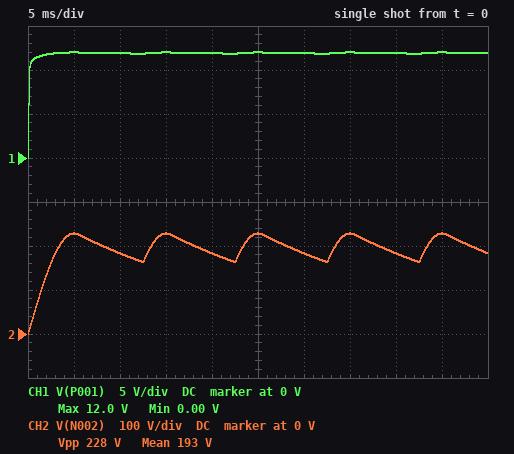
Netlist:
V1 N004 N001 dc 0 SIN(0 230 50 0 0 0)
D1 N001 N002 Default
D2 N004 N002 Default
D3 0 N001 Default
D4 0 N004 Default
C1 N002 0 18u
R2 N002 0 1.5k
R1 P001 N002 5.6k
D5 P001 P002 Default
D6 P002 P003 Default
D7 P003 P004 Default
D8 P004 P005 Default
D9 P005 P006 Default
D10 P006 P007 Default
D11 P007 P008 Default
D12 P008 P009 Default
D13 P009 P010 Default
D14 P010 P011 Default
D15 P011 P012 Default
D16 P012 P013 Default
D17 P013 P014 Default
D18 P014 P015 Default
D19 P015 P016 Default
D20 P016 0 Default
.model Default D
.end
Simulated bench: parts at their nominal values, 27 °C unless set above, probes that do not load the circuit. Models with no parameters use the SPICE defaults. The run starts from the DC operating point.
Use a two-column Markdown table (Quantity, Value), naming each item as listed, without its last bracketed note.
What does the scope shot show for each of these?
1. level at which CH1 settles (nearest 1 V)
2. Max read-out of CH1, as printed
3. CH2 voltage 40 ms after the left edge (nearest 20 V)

| Quantity | Value |
|---|---|
| level at which CH1 settles | 12 V |
| Max read-out of CH1, as printed | 12.0 V |
| CH2 voltage 40 ms after the left edge | 180 V |
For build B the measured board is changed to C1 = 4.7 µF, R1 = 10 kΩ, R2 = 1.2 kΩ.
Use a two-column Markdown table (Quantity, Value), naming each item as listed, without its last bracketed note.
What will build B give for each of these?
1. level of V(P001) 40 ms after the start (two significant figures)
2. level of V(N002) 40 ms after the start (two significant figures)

| Quantity | Value |
|---|---|
| level of V(P001) 40 ms after the start | 11 V |
| level of V(N002) 40 ms after the start | 100 V |
